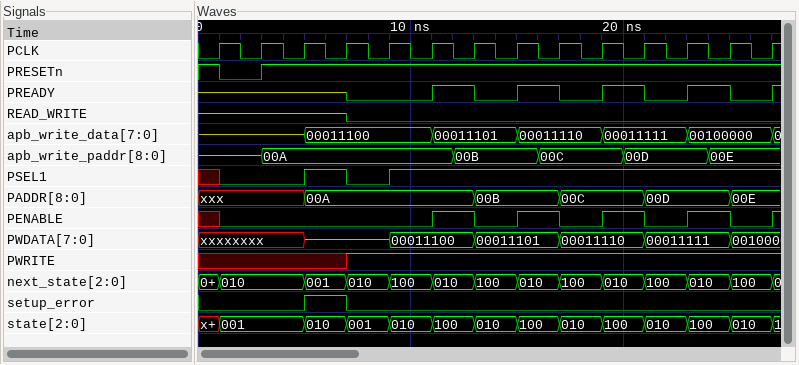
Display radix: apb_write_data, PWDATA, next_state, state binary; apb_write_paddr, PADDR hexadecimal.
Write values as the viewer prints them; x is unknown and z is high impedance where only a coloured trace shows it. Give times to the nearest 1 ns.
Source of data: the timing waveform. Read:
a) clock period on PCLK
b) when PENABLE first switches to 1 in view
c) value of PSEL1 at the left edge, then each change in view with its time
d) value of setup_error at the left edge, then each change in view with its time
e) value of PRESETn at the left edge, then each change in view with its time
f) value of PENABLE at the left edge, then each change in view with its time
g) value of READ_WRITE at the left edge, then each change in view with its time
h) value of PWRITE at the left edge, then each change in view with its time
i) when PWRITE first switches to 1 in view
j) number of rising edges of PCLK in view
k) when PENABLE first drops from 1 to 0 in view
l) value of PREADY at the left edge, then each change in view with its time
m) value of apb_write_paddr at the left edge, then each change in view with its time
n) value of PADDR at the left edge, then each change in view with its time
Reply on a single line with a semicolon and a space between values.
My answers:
2 ns; 11 ns; x, 0 at 1 ns, 1 at 5 ns, 0 at 7 ns, 1 at 9 ns; 0, 1 at 5 ns, 0 at 7 ns; 1, 0 at 1 ns, 1 at 3 ns; x, 0 at 1 ns, 1 at 11 ns, 0 at 13 ns, 1 at 15 ns, 0 at 17 ns, 1 at 19 ns, 0 at 21 ns, 1 at 23 ns, 0 at 25 ns, 1 at 27 ns; z, 0 at 7 ns; x, 1 at 7 ns; 7 ns; 14; 13 ns; z, 0 at 7 ns, 1 at 11 ns, 0 at 13 ns, 1 at 15 ns, 0 at 17 ns, 1 at 19 ns, 0 at 21 ns, 1 at 23 ns, 0 at 25 ns, 1 at 27 ns; z, 00A at 3 ns, 00B at 12 ns, 00C at 16 ns, 00D at 20 ns, 00E at 24 ns; xxx, 00A at 5 ns, 00B at 13 ns, 00C at 17 ns, 00D at 21 ns, 00E at 25 ns
